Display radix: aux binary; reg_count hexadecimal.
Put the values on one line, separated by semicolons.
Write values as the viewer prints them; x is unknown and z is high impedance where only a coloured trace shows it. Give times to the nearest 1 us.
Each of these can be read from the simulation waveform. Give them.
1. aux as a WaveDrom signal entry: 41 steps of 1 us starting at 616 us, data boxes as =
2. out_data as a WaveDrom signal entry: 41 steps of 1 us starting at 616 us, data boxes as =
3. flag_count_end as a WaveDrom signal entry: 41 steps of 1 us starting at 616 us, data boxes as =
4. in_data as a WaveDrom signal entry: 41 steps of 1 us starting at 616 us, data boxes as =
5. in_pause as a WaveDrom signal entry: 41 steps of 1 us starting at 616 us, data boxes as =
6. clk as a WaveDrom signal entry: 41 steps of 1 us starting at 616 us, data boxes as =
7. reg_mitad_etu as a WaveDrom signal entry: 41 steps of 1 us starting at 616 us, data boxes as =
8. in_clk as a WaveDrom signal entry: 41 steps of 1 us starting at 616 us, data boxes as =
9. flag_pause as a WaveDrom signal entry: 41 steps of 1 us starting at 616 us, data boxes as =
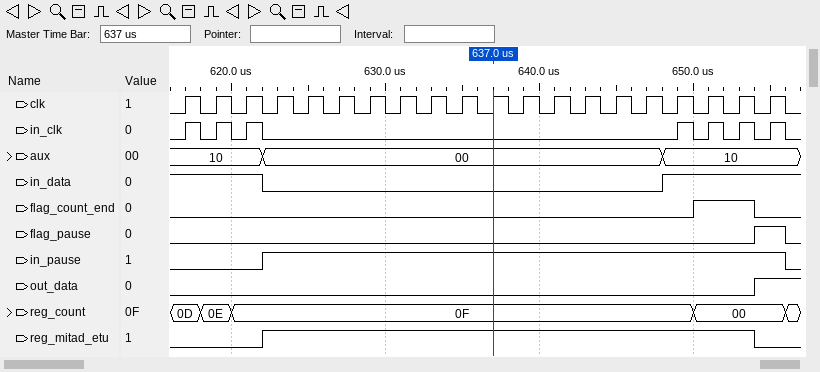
{name: 'aux', wave: '=.....=.........................=........', data: '10 00 10'}; {name: 'out_data', wave: '0.....................................1..'}; {name: 'flag_count_end', wave: '0.................................1...0..'}; {name: 'in_data', wave: '1.....0.........................1........'}; {name: 'in_pause', wave: '0.....1.................................0'}; {name: 'clk', wave: '01010101010101010101010101010101010101010'}; {name: 'reg_mitad_etu', wave: '0.....1...............................0..'}; {name: 'in_clk', wave: '0101010..........................10101010'}; {name: 'flag_pause', wave: '0.....................................1.0'}
